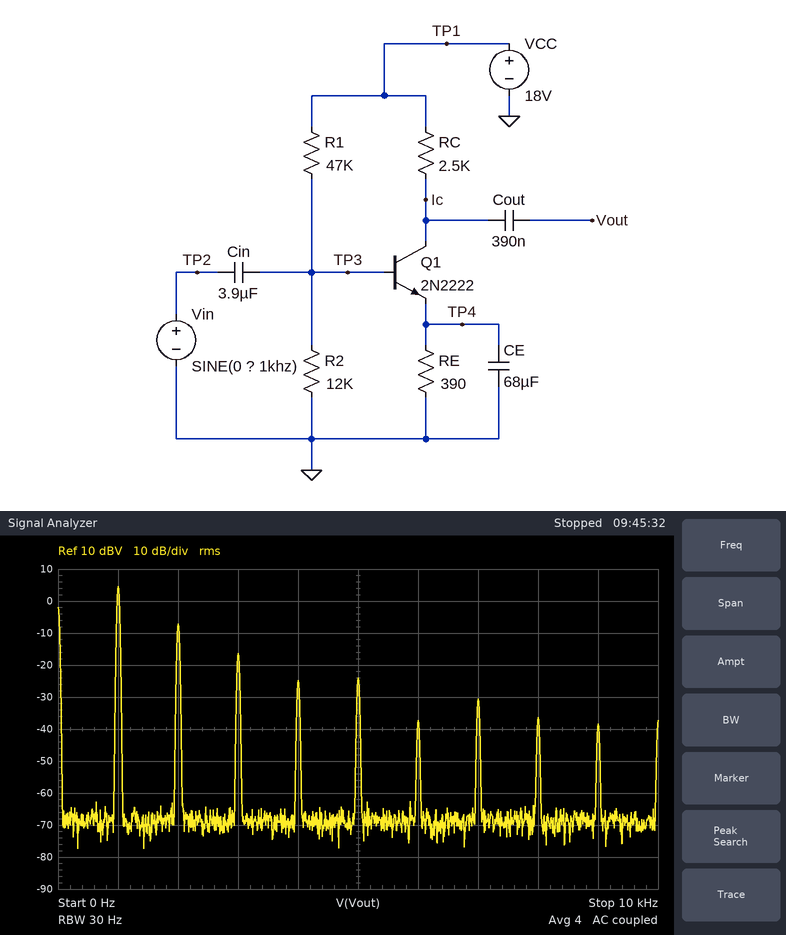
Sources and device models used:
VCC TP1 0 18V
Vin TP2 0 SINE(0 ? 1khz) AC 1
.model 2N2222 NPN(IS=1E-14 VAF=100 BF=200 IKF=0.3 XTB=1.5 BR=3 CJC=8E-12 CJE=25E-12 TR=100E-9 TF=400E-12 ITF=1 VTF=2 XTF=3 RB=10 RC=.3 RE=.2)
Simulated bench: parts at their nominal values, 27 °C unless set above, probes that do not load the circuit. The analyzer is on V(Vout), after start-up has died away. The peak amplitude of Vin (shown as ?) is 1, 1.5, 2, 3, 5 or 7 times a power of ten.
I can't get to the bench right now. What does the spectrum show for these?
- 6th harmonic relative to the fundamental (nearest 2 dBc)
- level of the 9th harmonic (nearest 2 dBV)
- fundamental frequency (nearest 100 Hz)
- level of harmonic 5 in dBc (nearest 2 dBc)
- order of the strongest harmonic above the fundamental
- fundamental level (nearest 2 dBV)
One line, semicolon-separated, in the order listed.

-42 dBc; -38 dBV; 1.0 kHz; -28 dBc; 2; 4 dBV
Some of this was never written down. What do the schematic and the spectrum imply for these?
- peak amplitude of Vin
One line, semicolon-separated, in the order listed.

10 mV
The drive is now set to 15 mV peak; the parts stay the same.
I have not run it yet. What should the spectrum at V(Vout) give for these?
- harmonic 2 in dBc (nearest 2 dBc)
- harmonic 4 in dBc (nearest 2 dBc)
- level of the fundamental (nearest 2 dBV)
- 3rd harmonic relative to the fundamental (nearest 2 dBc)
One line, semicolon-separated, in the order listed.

-14 dBc; -34 dBc; 8 dBV; -20 dBc
